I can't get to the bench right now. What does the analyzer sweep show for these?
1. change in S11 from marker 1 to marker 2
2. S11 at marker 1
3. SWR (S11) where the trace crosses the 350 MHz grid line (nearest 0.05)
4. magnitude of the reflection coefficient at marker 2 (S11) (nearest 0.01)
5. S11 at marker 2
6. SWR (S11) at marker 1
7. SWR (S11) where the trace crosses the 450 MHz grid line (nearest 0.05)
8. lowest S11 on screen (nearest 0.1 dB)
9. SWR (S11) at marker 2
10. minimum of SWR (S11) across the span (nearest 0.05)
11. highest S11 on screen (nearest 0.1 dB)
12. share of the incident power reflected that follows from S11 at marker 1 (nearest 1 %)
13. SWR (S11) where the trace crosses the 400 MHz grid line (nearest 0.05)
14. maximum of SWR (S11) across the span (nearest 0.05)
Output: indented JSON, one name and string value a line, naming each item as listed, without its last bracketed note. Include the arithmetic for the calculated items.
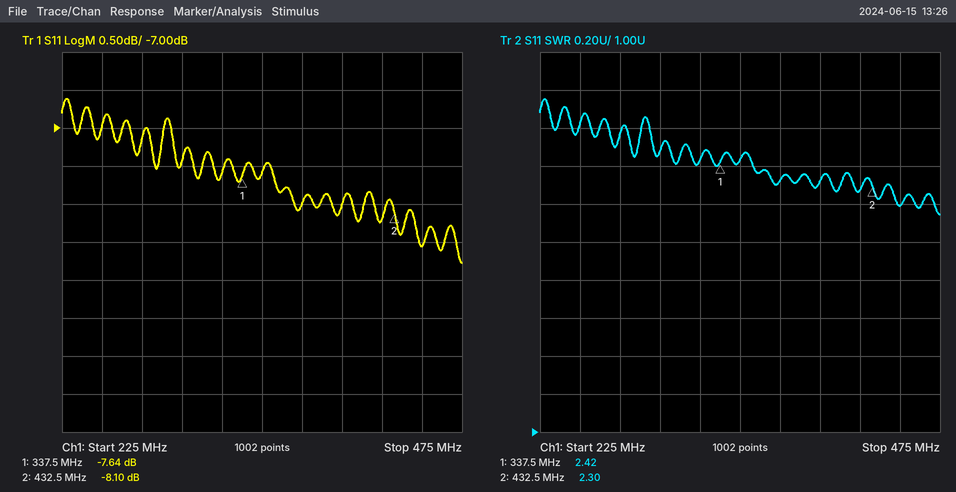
{
  "change in S11 from marker 1 to marker 2": "-8.1 − (-7.64) = -0.46 dB",
  "S11 at marker 1": "-7.64 dB",
  "SWR (S11) where the trace crosses the 350 MHz grid line": "2.45",
  "magnitude of the reflection coefficient at marker 2 (S11)": "10^(-8.1/20) ≈ 0.39",
  "S11 at marker 2": "-8.10 dB",
  "SWR (S11) at marker 1": "2.42",
  "SWR (S11) where the trace crosses the 450 MHz grid line": "2.20",
  "lowest S11 on screen": "-8.8 dB",
  "SWR (S11) at marker 2": "2.30",
  "minimum of SWR (S11) across the span": "2.15",
  "highest S11 on screen": "-6.6 dB",
  "share of the incident power reflected that follows from S11 at marker 1": "10^(-7.64/10) ≈ 17 %",
  "SWR (S11) where the trace crosses the 400 MHz grid line": "2.30",
  "maximum of SWR (S11) across the span": "2.75"
}
